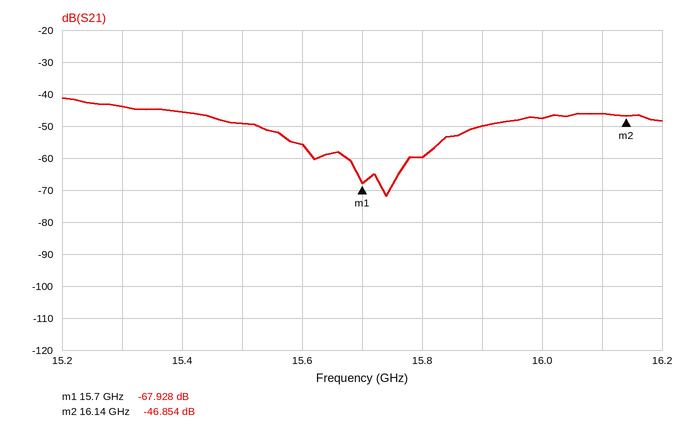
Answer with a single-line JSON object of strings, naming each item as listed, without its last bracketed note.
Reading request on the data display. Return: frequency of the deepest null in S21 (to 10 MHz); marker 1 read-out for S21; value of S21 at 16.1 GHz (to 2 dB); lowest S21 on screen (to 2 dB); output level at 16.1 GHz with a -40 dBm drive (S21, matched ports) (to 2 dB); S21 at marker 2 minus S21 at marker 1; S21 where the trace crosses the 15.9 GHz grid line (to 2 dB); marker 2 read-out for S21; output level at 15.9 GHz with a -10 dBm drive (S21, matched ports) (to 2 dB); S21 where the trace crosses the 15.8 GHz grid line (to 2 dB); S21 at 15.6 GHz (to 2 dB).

{"frequency of the deepest null in S21": "15.74 GHz", "marker 1 read-out for S21": "-67.928 dB", "value of S21 at 16.1 GHz": "-46 dB", "lowest S21 on screen": "-72 dB", "output level at 16.1 GHz with a -40 dBm drive (S21, matched ports)": "-86 dBm", "S21 at marker 2 minus S21 at marker 1": "21.074 dB", "S21 where the trace crosses the 15.9 GHz grid line": "-50 dB", "marker 2 read-out for S21": "-46.854 dB", "output level at 15.9 GHz with a -10 dBm drive (S21, matched ports)": "-60 dBm", "S21 where the trace crosses the 15.8 GHz grid line": "-60 dB", "S21 at 15.6 GHz": "-56 dB"}
